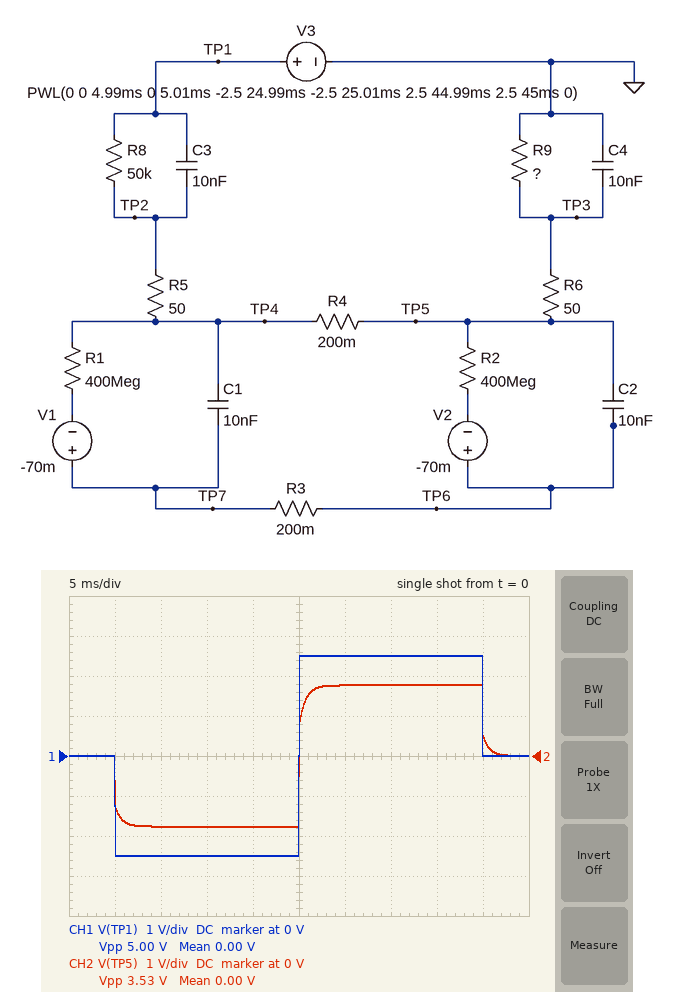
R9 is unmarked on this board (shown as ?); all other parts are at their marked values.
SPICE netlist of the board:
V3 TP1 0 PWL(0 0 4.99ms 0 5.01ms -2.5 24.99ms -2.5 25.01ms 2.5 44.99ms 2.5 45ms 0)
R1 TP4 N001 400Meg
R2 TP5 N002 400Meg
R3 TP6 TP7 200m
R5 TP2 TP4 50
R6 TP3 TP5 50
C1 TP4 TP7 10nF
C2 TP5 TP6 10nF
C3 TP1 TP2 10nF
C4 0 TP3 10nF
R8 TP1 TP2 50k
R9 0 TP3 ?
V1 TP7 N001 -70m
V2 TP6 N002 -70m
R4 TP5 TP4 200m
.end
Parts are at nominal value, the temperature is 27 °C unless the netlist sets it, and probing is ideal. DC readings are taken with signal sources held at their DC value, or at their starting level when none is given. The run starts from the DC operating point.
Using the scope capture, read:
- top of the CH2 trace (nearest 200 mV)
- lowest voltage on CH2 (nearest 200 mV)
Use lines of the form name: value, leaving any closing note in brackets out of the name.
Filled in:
top of the CH2 trace: 1.8 V
lowest voltage on CH2: -1.8 V
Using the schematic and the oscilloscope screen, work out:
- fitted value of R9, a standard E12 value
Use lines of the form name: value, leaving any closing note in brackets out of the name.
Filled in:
fitted value of R9, a standard E12 value: 120 kΩ
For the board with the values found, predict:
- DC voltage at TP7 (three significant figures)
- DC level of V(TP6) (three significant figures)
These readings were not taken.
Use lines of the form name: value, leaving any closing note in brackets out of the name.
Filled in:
DC voltage at TP7: -70.0 mV
DC level of V(TP6): -70.0 mV
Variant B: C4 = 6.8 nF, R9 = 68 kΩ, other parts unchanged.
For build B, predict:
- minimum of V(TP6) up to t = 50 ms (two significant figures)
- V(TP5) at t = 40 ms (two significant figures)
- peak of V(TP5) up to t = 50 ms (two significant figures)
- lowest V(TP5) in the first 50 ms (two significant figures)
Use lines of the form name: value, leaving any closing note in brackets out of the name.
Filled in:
minimum of V(TP6) up to t = 50 ms: -1.6 V
V(TP5) at t = 40 ms: 1.4 V
peak of V(TP5) up to t = 50 ms: 1.5 V
lowest V(TP5) in the first 50 ms: -1.5 V
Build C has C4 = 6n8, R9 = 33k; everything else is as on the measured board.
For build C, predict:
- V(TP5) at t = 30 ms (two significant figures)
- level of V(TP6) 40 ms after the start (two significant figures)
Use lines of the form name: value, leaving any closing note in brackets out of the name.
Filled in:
V(TP5) at t = 30 ms: 990 mV
level of V(TP6) 40 ms after the start: 920 mV
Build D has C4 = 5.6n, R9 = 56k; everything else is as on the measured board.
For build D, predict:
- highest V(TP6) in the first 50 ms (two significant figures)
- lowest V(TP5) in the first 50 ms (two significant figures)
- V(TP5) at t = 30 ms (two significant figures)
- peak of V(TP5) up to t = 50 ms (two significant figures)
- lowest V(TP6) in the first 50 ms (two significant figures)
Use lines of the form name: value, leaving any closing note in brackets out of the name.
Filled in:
highest V(TP6) in the first 50 ms: 1.8 V
lowest V(TP5) in the first 50 ms: -1.6 V
V(TP5) at t = 30 ms: 1.3 V
peak of V(TP5) up to t = 50 ms: 1.9 V
lowest V(TP6) in the first 50 ms: -1.7 V
